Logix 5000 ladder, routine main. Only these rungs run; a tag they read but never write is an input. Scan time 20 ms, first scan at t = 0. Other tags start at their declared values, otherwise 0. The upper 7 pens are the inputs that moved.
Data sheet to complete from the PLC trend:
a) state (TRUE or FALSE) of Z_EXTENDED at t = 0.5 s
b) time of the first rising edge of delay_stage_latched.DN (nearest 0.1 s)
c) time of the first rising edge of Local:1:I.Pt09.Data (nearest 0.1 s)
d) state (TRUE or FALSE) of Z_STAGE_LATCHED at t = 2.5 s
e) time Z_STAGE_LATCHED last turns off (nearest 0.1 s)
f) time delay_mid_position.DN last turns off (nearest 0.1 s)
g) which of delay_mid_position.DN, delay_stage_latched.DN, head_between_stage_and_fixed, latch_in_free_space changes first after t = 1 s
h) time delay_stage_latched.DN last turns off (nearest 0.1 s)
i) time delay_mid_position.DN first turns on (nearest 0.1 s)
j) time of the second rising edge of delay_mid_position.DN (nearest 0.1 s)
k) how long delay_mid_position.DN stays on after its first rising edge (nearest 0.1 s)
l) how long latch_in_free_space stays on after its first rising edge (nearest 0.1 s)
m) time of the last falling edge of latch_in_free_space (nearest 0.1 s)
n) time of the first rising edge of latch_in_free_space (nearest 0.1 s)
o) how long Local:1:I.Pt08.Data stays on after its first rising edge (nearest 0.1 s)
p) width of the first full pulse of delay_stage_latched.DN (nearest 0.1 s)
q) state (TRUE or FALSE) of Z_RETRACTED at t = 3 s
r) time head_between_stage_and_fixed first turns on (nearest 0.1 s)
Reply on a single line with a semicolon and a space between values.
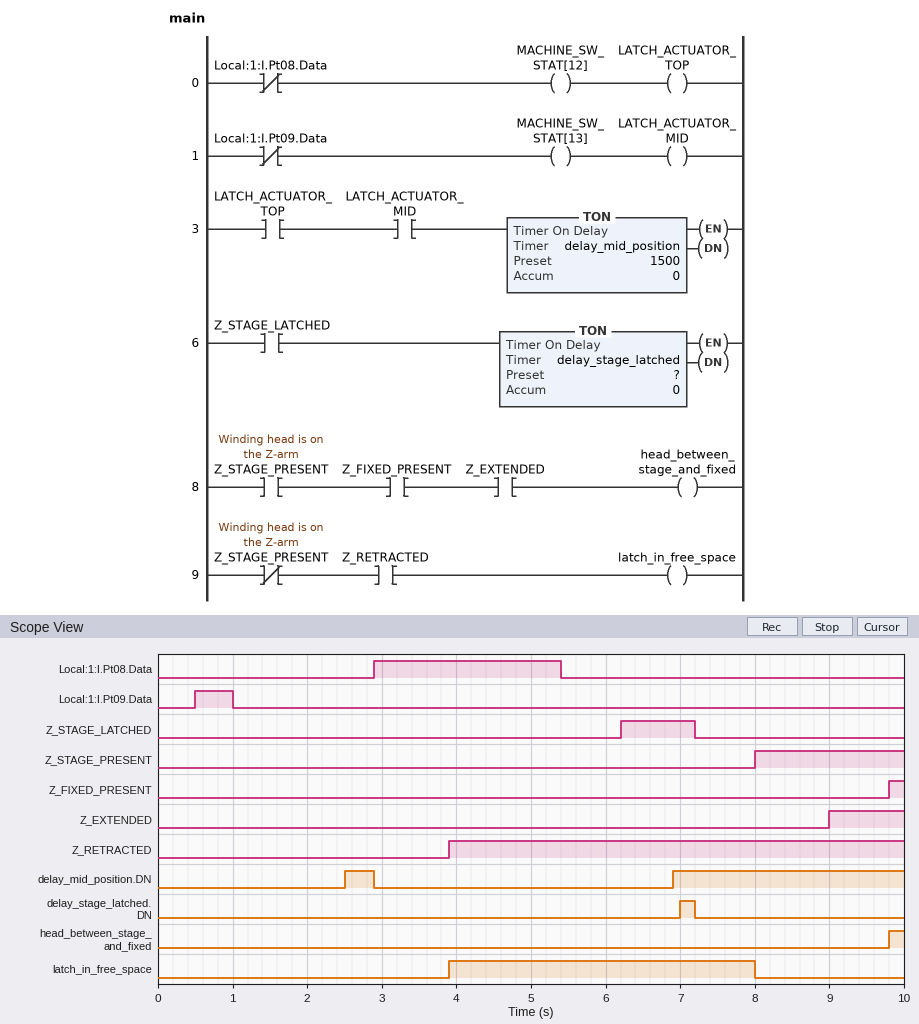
FALSE; 7.0 s; 0.5 s; FALSE; 7.2 s; 2.9 s; delay_mid_position.DN; 7.2 s; 2.5 s; 6.9 s; 0.4 s; 4.1 s; 8.0 s; 3.9 s; 2.5 s; 0.2 s; FALSE; 9.8 s
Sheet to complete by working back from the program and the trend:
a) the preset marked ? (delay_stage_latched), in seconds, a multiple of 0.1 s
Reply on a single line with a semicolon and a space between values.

0.8 s
